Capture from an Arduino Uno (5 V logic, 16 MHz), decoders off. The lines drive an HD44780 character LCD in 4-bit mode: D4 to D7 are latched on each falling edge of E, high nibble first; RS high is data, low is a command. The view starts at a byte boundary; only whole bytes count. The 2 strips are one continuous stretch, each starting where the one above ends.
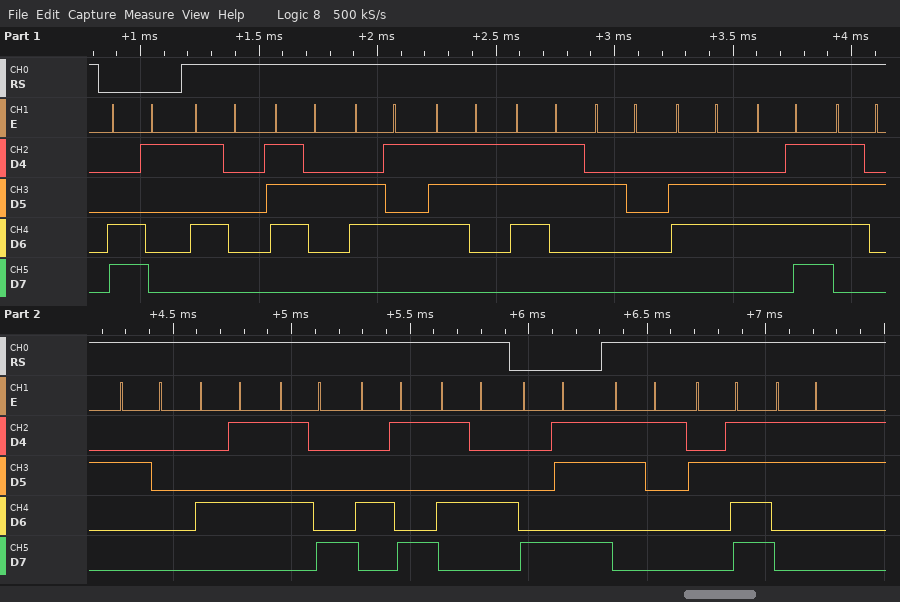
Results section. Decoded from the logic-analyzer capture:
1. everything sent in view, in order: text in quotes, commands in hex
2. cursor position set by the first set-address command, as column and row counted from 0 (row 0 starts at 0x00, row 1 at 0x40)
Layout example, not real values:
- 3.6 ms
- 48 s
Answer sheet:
- 0xC1 "Press for EXIT" 0x8B "1/3"
- column 1, row 1
